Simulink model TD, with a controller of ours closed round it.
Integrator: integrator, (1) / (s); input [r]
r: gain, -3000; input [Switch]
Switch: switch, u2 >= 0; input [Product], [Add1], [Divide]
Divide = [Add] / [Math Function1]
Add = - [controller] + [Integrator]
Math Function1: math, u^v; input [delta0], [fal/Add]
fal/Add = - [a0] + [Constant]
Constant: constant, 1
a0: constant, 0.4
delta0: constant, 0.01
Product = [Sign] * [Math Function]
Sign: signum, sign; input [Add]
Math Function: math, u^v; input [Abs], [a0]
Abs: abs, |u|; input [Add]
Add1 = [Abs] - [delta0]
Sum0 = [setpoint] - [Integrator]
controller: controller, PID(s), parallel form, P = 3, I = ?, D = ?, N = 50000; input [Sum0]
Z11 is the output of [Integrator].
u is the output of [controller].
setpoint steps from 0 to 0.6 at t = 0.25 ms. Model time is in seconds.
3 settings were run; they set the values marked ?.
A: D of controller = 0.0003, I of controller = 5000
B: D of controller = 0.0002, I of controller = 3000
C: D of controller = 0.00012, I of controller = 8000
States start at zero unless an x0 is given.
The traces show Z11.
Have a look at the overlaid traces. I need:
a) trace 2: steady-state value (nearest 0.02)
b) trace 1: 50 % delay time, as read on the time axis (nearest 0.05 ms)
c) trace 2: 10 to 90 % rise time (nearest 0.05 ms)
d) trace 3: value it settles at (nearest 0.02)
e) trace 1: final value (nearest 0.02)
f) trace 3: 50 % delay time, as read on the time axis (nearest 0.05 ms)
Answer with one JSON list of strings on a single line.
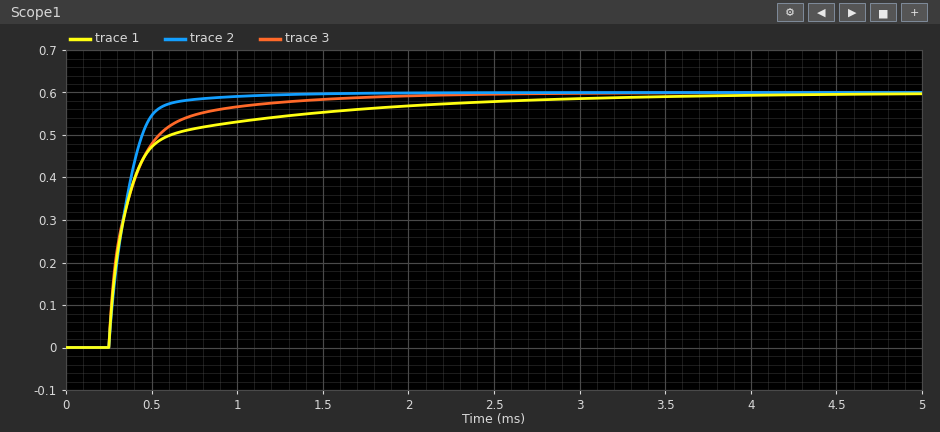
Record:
["0.60", "0.35 ms", "0.25 ms", "0.60", "0.60", "0.35 ms"]
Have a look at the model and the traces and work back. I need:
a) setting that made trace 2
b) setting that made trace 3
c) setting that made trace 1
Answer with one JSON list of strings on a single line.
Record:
["C", "A", "B"]
